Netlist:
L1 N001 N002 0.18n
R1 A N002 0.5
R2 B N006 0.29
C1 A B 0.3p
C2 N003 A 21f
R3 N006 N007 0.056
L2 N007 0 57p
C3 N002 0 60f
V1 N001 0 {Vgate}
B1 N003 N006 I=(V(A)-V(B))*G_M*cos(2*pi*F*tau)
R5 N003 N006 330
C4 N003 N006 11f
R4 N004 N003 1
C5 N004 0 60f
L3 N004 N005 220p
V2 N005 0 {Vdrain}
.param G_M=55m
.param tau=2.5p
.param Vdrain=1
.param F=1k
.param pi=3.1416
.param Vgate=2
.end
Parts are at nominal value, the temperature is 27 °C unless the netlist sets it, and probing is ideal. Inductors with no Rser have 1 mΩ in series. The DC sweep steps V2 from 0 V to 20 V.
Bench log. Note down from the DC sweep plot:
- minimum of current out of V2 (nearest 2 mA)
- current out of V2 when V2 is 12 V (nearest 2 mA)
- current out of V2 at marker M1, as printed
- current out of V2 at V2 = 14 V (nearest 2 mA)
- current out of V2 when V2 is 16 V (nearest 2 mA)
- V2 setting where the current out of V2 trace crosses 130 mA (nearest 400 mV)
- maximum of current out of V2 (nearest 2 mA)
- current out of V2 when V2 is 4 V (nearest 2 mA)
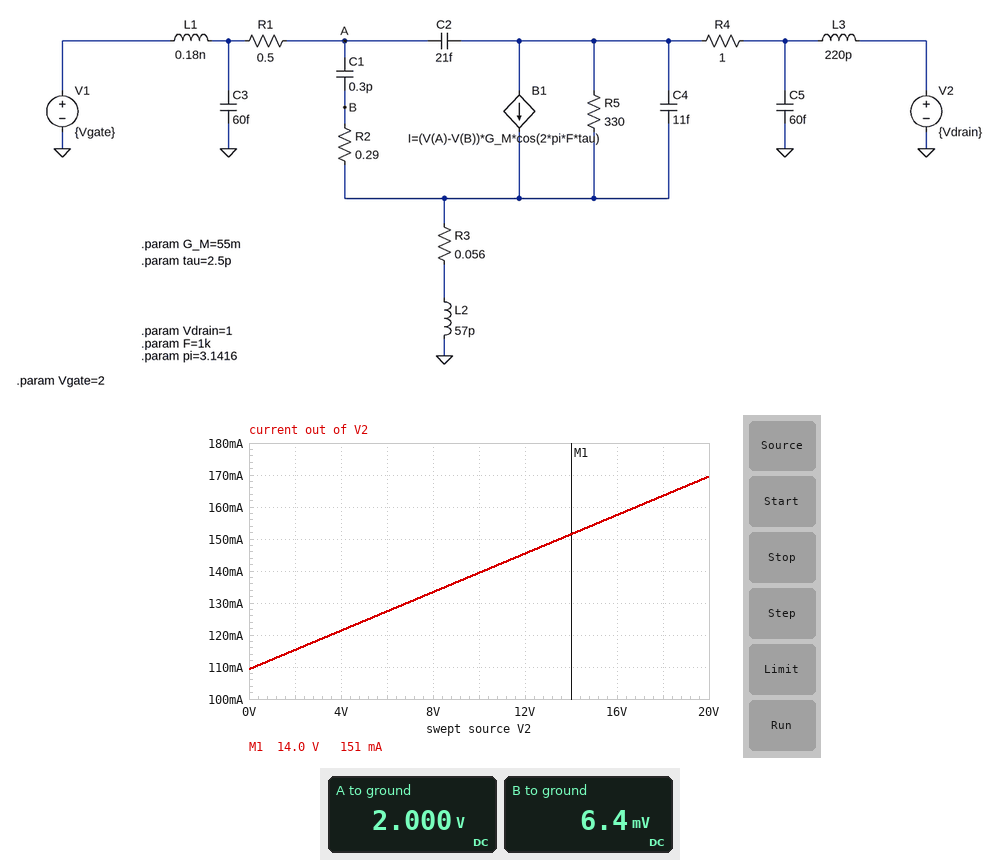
110 mA
146 mA
151 mA
152 mA
158 mA
6.8 V
170 mA
122 mA
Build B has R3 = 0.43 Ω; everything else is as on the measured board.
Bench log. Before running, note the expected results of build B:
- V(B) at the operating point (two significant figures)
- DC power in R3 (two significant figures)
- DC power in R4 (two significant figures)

47 mV
5.2 mW
12 mW
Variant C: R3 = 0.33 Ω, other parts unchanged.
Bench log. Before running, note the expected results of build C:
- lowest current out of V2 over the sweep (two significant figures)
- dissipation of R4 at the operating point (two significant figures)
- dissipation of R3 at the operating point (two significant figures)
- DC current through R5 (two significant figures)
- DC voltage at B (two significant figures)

110 mA
12 mW
4.0 mW
2.6 mA
37 mV
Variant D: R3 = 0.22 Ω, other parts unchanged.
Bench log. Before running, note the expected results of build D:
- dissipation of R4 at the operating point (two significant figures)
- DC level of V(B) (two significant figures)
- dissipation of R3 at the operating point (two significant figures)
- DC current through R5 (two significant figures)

12 mW
25 mV
2.7 mW
2.6 mA
